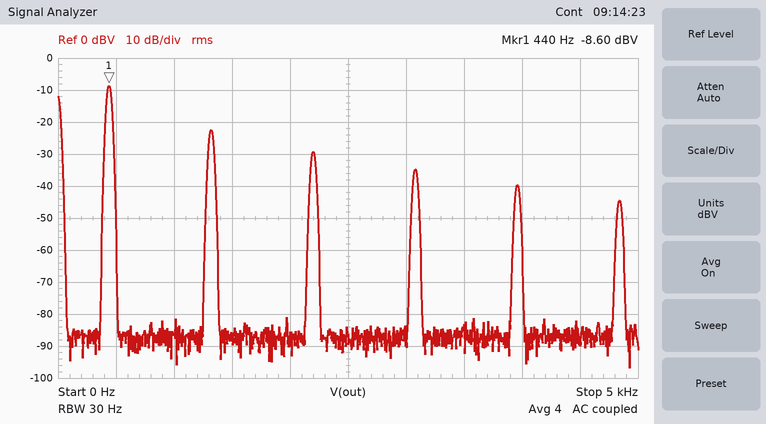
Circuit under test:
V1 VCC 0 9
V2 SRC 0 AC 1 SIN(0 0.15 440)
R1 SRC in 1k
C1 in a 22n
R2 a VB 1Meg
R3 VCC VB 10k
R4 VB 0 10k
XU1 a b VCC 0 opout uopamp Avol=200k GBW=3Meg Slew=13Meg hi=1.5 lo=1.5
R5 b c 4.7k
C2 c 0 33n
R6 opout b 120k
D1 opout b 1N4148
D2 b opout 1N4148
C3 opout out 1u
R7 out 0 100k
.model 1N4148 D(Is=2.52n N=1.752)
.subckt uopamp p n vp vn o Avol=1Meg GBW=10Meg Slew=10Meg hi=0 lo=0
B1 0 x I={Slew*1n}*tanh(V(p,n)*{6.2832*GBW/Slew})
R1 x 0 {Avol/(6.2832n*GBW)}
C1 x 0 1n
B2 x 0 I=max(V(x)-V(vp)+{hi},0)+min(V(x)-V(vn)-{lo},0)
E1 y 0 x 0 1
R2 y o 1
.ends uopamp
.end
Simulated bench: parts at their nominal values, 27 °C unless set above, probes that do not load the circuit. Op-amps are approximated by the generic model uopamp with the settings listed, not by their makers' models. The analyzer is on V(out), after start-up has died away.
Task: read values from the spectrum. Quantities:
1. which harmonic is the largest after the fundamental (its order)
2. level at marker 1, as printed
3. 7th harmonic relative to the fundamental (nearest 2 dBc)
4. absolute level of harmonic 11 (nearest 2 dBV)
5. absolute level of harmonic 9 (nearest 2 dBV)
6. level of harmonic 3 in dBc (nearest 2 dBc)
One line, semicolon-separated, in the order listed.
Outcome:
3; -8.60 dBV; -26 dBc; -44 dBV; -40 dBV; -14 dBc
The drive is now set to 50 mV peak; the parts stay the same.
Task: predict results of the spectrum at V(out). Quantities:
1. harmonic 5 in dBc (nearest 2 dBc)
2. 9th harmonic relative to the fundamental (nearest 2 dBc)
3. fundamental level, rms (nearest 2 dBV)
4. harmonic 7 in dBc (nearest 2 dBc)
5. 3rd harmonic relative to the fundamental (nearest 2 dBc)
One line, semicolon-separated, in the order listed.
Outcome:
-32 dBc; -54 dBc; -12 dBV; -58 dBc; -18 dBc
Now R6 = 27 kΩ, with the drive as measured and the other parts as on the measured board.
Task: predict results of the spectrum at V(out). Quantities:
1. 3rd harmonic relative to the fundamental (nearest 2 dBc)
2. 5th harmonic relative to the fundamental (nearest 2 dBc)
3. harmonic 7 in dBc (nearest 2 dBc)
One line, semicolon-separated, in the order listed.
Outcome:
-30 dBc; -48 dBc; -60 dBc
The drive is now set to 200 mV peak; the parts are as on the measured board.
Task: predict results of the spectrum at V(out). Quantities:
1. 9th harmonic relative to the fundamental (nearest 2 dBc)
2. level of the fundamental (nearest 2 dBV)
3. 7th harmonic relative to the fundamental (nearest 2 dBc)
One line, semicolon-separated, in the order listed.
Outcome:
-28 dBc; -8 dBV; -24 dBc
